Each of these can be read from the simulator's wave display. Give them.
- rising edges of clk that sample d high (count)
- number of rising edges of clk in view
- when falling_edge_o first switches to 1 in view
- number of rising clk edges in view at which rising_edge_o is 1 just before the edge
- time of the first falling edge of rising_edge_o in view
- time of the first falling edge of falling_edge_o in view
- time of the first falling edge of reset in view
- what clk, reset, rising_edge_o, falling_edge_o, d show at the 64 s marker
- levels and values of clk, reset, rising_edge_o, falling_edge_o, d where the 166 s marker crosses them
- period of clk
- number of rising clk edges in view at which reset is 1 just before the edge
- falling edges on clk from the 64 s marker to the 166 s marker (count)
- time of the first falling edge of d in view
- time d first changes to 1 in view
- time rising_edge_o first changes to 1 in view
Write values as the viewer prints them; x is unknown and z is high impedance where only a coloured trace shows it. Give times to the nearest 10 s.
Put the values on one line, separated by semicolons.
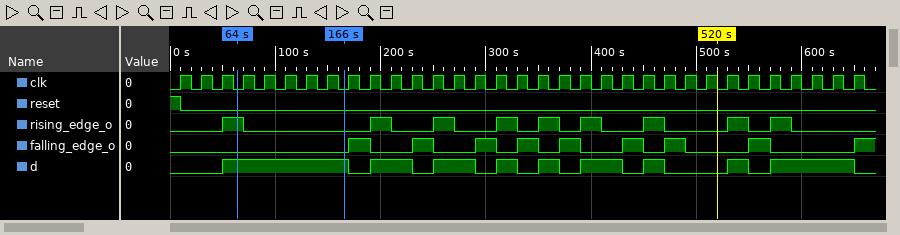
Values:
20; 33; 170 s; 9; 70 s; 190 s; 10 s; clk=0, reset=0, rising_edge_o=1, falling_edge_o=0, d=1; clk=0, reset=0, rising_edge_o=0, falling_edge_o=0, d=1; 20 s; 1; 5; 170 s; 50 s; 50 s
